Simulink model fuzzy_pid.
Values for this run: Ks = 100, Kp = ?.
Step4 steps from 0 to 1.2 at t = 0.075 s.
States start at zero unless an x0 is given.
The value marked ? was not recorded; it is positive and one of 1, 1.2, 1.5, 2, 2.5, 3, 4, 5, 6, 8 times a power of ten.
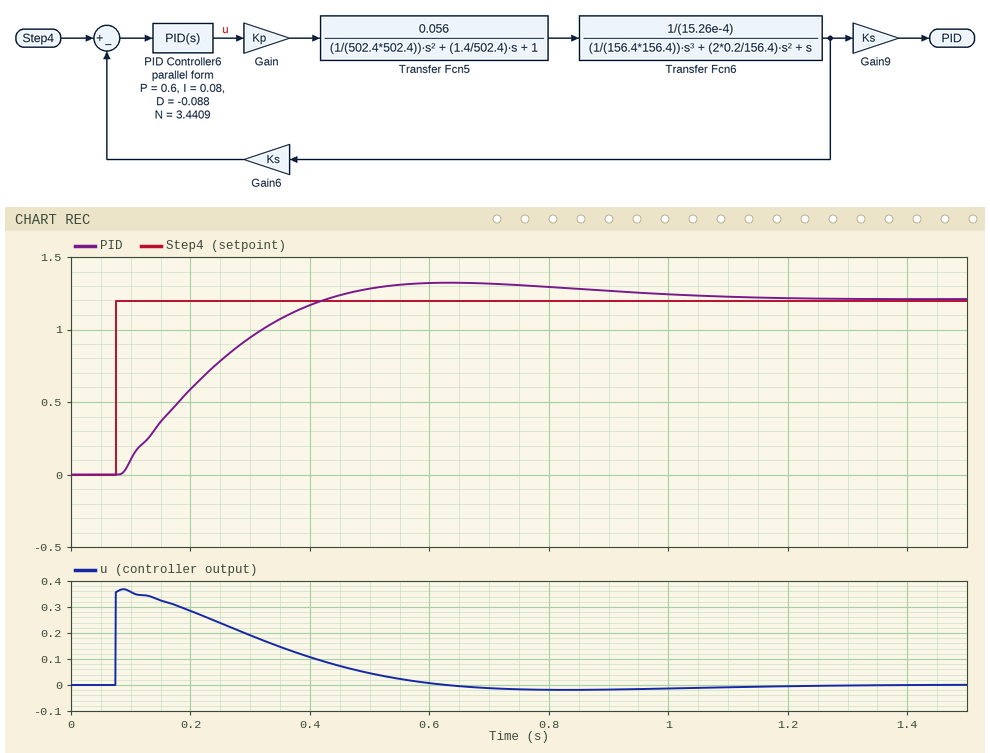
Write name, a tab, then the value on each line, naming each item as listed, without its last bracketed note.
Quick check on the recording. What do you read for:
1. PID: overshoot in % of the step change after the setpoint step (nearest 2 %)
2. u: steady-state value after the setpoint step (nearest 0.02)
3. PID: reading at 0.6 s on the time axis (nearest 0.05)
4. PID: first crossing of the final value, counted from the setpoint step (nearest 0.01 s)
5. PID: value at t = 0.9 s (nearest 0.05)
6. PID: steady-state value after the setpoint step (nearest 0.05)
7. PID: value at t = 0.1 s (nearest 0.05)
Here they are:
PID: overshoot in % of the step change after the setpoint step	10 %
u: steady-state value after the setpoint step	0.00
PID: reading at 0.6 s on the time axis	1.30
PID: first crossing of the final value, counted from the setpoint step	0.35 s
PID: value at t = 0.9 s	1.25
PID: steady-state value after the setpoint step	1.20
PID: value at t = 0.1 s	0.10
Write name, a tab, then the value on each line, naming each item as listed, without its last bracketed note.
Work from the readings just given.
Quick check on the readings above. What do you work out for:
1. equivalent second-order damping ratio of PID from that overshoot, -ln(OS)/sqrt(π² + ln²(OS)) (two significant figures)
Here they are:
equivalent second-order damping ratio of PID from that overshoot, -ln(OS)/sqrt(π² + ln²(OS))	0.59
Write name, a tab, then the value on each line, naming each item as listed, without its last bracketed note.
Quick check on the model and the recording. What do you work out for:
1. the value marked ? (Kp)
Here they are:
the value marked ?	0.004
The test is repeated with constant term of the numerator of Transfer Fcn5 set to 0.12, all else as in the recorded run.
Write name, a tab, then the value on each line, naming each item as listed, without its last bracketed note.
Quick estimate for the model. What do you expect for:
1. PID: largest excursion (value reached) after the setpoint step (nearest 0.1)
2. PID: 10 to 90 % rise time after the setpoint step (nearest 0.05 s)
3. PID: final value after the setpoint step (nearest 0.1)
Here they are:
PID: largest excursion (value reached) after the setpoint step	1.3
PID: 10 to 90 % rise time after the setpoint step	0.15 s
PID: final value after the setpoint step	1.2
